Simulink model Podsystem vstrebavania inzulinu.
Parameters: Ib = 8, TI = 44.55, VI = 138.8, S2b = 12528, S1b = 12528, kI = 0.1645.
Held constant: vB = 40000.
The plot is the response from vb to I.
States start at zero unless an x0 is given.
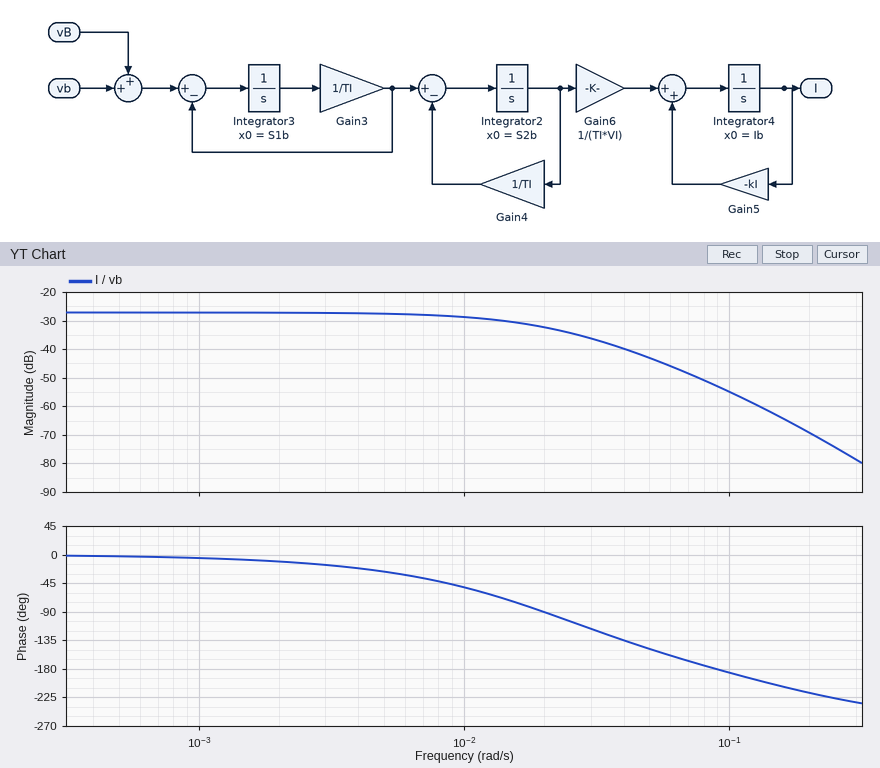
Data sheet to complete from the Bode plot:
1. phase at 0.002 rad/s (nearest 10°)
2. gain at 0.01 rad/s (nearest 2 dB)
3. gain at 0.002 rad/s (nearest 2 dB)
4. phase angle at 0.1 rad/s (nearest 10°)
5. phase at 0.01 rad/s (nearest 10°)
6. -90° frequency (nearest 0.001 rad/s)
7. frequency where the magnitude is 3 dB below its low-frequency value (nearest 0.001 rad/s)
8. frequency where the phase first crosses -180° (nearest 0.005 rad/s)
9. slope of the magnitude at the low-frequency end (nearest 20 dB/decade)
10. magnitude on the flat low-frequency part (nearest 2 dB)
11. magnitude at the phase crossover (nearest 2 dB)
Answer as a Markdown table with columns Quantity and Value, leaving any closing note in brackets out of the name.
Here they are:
| Quantity | Value |
|---|---|
| phase at 0.002 rad/s | -10° |
| gain at 0.01 rad/s | -28 dB |
| gain at 0.002 rad/s | -28 dB |
| phase angle at 0.1 rad/s | -190° |
| phase at 0.01 rad/s | -50° |
| -90° frequency | 0.020 rad/s |
| frequency where the magnitude is 3 dB below its low-frequency value | 0.014 rad/s |
| frequency where the phase first crosses -180° | 0.090 rad/s |
| slope of the magnitude at the low-frequency end | 0 dB/decade |
| magnitude on the flat low-frequency part | -28 dB |
| magnitude at the phase crossover | -52 dB |
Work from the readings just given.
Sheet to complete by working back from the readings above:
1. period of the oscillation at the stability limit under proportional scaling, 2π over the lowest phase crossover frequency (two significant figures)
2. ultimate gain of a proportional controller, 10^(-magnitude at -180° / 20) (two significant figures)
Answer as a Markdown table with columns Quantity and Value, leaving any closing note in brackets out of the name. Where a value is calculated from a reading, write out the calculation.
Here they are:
| Quantity | Value |
|---|---|
| period of the oscillation at the stability limit under proportional scaling, 2π over the lowest phase crossover frequency | 2π / 0.09 = 70 s |
| ultimate gain of a proportional controller, 10^(-magnitude at -180° / 20) | 10^(52 / 20) = 400 |
